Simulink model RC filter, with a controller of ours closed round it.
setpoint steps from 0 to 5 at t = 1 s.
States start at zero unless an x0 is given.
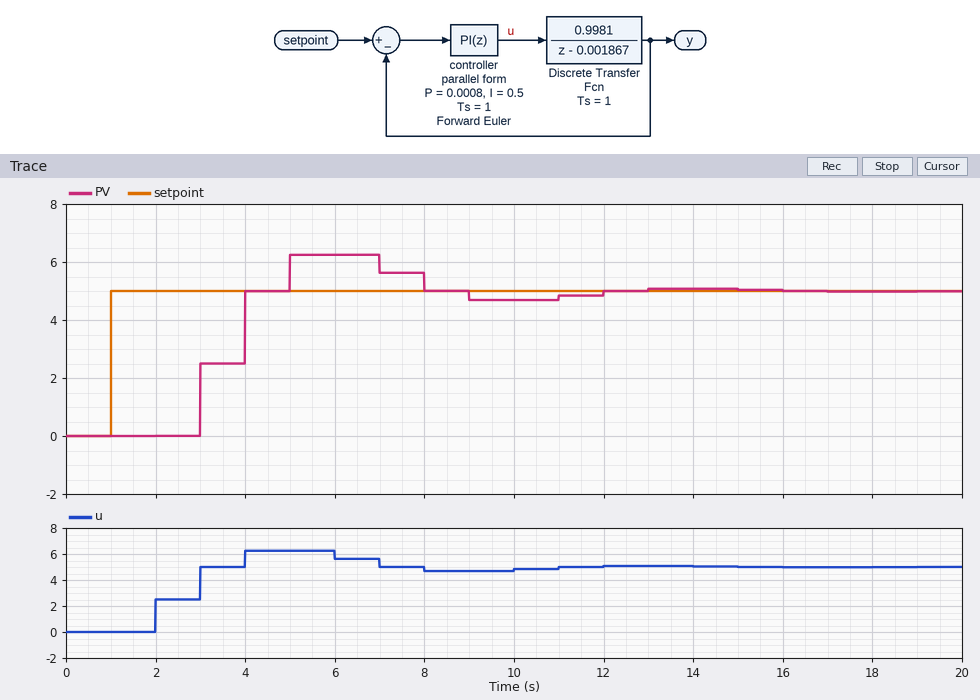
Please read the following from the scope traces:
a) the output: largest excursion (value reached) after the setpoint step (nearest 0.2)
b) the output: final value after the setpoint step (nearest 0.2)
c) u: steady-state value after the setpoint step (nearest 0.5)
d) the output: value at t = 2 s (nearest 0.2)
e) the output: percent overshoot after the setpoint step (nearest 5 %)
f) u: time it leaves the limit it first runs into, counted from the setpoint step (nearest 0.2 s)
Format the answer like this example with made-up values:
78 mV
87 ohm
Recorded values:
6.2
5.0
5.0
0.0
25 %
1.0 s
